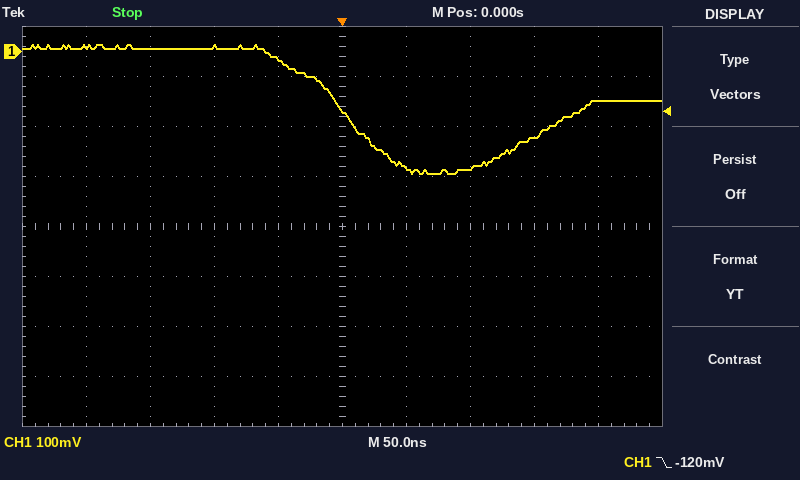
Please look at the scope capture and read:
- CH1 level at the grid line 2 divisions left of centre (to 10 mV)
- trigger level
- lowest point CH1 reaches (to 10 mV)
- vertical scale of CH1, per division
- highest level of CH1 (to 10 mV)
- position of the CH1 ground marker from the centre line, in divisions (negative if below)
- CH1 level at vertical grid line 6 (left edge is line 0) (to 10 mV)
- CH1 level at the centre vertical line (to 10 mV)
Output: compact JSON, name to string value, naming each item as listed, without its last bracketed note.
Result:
{"CH1 level at the grid line 2 divisions left of centre": "10 mV", "trigger level": "-120 mV", "lowest point CH1 reaches": "-240 mV", "vertical scale of CH1, per division": "100 mV", "highest level of CH1": "10 mV", "position of the CH1 ground marker from the centre line, in divisions": "+3.5 div", "CH1 level at vertical grid line 6 (left edge is line 0)": "-230 mV", "CH1 level at the centre vertical line": "-120 mV"}
